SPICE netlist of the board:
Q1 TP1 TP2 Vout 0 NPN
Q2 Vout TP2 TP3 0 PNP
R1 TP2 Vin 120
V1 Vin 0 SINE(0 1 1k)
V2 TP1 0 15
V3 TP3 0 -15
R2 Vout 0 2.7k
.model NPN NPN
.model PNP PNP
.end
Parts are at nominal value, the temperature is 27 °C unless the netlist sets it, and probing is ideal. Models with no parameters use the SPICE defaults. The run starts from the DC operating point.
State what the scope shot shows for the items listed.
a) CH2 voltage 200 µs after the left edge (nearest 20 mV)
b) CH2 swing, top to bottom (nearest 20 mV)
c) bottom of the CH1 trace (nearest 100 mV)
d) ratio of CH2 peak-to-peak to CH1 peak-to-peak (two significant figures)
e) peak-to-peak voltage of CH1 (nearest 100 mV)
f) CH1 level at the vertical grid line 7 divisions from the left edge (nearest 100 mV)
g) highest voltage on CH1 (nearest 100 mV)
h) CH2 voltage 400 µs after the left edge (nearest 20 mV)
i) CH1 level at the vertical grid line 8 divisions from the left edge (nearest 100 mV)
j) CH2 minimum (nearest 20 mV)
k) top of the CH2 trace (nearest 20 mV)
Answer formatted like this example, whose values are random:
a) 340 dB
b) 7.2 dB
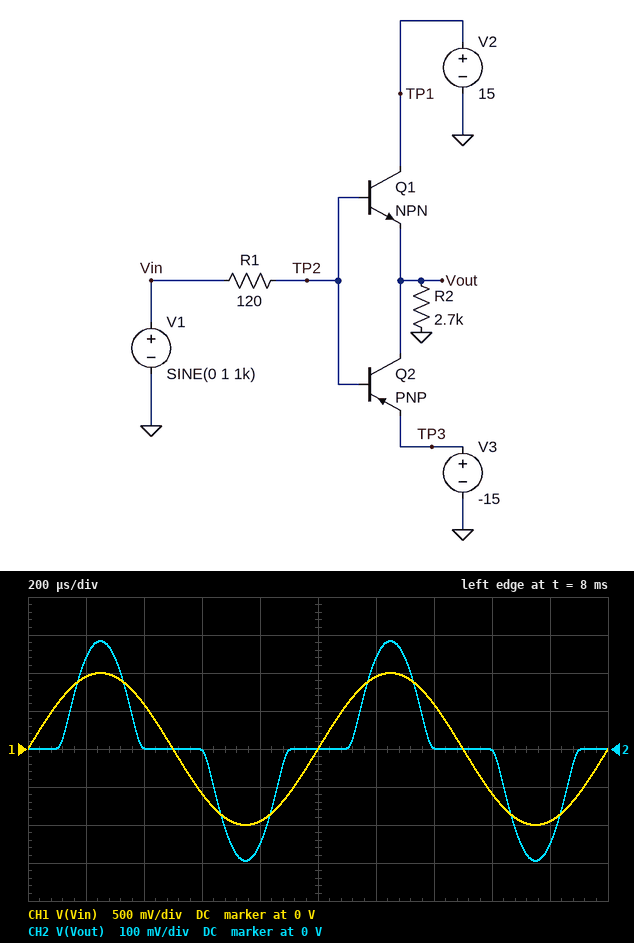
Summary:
a) 240 mV
b) 580 mV
c) -1.0 V
d) 0.29
e) 2.0 V
f) 600 mV
g) 1.0 V
h) 0 V
i) -600 mV
j) -300 mV
k) 280 mV
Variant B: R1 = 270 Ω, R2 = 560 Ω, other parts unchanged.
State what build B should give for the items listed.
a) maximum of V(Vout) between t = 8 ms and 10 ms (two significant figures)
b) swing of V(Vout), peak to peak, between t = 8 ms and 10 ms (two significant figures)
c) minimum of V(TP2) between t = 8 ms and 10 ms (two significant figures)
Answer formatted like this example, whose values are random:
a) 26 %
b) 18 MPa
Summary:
a) 250 mV
b) 460 mV
c) -950 mV
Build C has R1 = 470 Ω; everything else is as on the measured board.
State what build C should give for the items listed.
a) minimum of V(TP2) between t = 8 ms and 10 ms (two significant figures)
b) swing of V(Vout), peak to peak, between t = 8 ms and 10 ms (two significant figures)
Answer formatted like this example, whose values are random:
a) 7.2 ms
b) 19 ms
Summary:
a) -980 mV
b) 560 mV
